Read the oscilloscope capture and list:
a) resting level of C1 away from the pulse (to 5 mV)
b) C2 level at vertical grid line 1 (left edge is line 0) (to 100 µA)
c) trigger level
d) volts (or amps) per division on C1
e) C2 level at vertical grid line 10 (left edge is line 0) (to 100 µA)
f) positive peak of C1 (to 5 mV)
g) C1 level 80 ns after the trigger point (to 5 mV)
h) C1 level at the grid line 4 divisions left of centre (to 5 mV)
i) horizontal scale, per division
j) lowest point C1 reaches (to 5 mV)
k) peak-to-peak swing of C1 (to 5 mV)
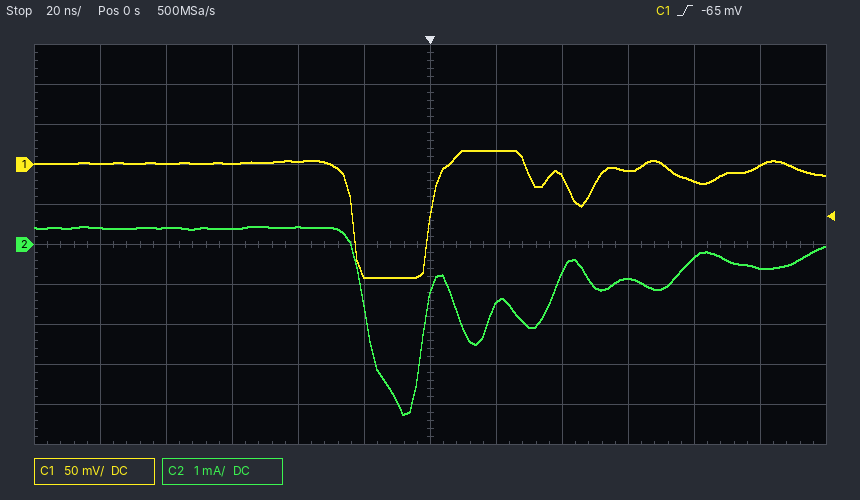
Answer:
0 mV
400 µA
-65 mV
50 mV
-300 µA
20 mV
-20 mV
0 mV
20 ns
-140 mV
160 mV
